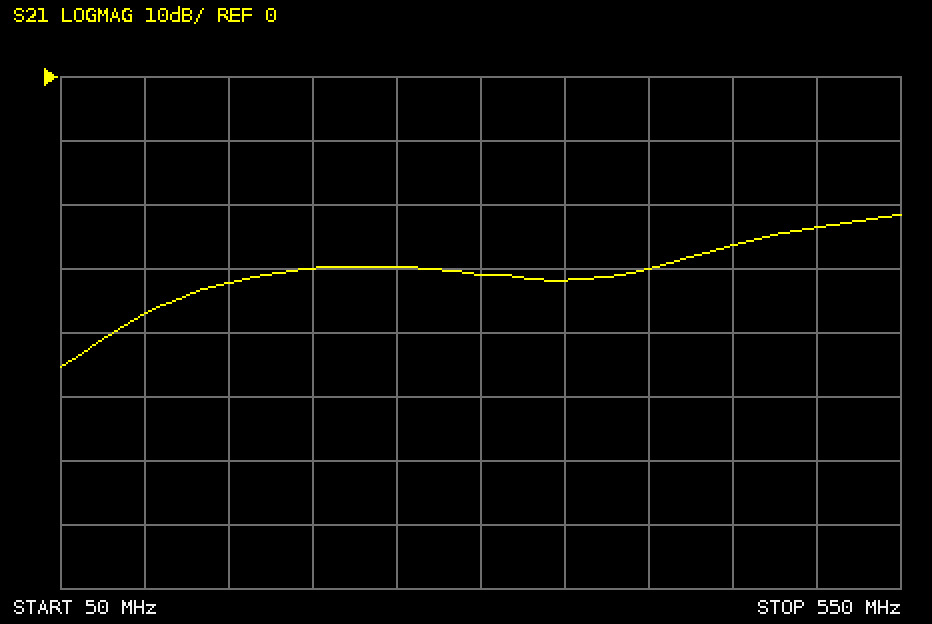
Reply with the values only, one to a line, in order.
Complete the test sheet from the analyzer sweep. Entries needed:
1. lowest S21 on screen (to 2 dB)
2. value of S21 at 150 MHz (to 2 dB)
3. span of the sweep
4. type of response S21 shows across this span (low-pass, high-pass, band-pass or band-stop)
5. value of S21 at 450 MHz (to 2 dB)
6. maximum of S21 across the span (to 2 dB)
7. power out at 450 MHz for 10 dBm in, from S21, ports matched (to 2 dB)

-46 dB
-32 dB
500 MHz
high-pass
-26 dB
-22 dB
-16 dBm
